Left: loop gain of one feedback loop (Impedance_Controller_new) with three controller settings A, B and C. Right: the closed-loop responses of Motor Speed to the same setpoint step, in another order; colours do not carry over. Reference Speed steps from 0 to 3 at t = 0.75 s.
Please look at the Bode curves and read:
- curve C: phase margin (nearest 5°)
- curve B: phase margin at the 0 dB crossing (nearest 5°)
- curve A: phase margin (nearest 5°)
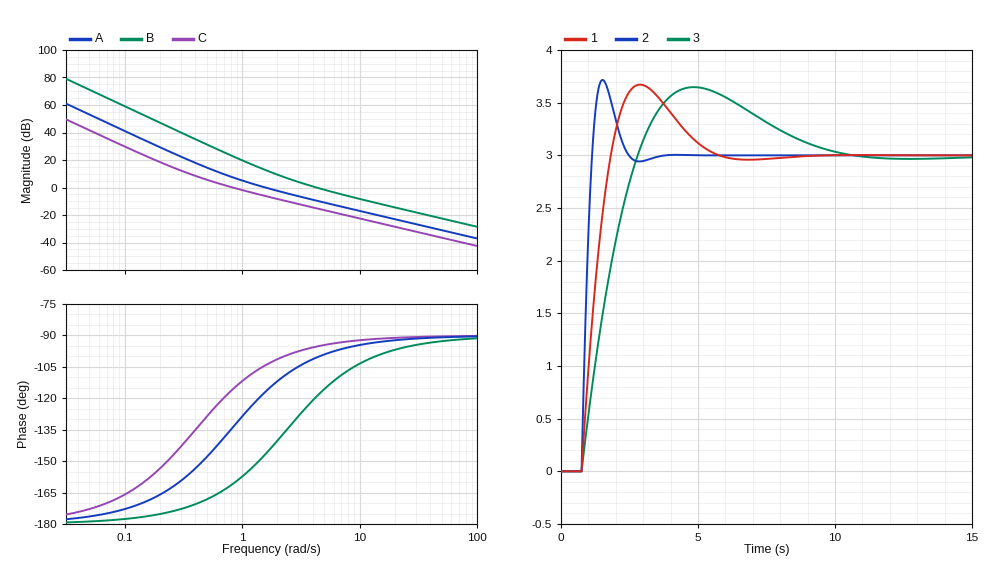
65°
60°
65°
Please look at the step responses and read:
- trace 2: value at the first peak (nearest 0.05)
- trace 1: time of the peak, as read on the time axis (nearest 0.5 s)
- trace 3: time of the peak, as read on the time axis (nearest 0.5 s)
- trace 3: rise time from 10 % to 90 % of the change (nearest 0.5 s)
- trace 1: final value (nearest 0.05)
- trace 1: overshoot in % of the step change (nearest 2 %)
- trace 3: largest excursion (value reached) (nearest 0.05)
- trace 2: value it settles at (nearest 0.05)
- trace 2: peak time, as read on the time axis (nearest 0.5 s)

3.70
3.0 s
5.0 s
1.5 s
3.00
22 %
3.65
3.00
1.5 s
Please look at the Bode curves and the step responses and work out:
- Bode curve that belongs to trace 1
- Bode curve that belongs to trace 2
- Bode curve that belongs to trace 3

A
B
C
